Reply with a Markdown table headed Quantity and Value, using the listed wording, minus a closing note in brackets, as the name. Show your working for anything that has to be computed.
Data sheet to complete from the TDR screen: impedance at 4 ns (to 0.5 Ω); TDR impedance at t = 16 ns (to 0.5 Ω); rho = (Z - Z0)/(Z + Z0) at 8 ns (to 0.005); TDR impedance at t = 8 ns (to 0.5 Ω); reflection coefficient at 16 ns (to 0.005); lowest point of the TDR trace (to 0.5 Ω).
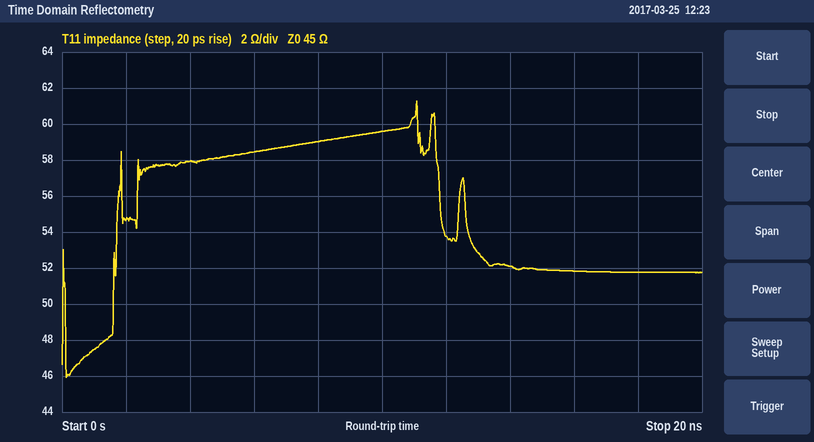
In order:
| Quantity | Value |
|---|---|
| impedance at 4 ns | 58.0 Ω |
| TDR impedance at t = 16 ns | 52.0 Ω |
| rho = (Z - Z0)/(Z + Z0) at 8 ns | (59 − 45)/(59 + 45) ≈ +0.135 |
| TDR impedance at t = 8 ns | 59.0 Ω |
| reflection coefficient at 16 ns | (52 − 45)/(52 + 45) ≈ +0.0722, so +0.070 to the nearest 0.005 |
| lowest point of the TDR trace | 46.0 Ω |
